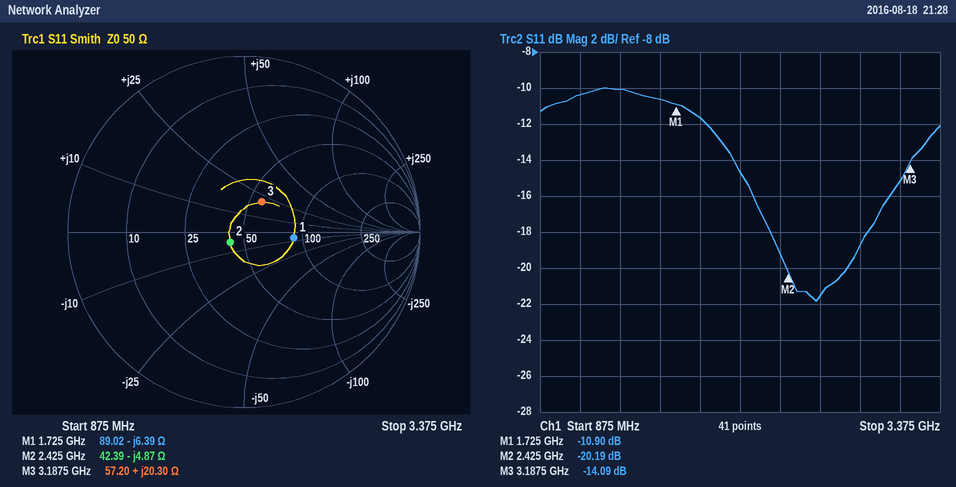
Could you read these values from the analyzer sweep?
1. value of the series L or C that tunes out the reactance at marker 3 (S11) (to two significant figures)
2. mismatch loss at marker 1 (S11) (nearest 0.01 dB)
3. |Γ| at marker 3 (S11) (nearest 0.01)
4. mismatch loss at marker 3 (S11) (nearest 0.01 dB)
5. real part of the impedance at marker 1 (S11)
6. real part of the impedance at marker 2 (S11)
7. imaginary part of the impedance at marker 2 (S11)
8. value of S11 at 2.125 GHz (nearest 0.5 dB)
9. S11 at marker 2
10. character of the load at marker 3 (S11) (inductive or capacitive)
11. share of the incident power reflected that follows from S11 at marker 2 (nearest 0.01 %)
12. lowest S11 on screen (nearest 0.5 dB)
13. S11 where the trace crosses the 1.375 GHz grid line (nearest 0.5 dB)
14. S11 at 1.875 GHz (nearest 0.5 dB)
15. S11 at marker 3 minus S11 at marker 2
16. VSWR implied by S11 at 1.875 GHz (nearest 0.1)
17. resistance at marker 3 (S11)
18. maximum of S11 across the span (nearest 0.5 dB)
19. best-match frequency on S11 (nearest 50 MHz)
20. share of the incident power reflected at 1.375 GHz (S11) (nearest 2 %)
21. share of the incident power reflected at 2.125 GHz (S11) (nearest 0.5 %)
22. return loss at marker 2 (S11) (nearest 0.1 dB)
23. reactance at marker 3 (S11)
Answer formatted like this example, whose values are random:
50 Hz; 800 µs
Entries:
2.5 pF; 0.37 dB; 0.20; 0.17 dB; 89.02 Ω; 42.39 Ω; -4.87 Ω; -14.5 dB; -20.19 dB; inductive; 0.96 %; -22.0 dB; -10.0 dB; -11.5 dB; 6.10 dB; 1.7; 57.20 Ω; -10.0 dB; 2.60 GHz; 10 %; 3.5 %; 20.2 dB; +20.30 Ω
